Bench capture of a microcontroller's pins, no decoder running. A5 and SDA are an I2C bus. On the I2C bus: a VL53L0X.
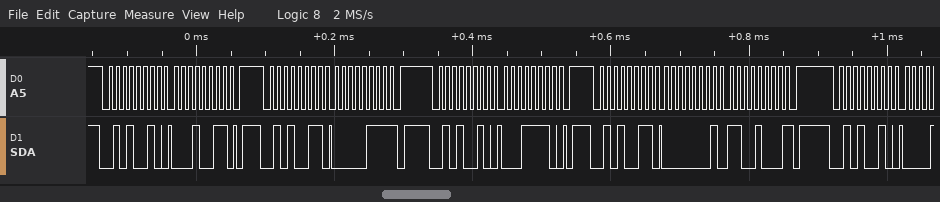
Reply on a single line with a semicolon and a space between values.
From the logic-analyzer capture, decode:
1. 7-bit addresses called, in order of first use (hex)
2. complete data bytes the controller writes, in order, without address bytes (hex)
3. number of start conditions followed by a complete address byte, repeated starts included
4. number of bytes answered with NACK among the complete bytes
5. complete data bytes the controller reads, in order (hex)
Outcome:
0x29; 13 1E; 5; 2; 07 01 C8
